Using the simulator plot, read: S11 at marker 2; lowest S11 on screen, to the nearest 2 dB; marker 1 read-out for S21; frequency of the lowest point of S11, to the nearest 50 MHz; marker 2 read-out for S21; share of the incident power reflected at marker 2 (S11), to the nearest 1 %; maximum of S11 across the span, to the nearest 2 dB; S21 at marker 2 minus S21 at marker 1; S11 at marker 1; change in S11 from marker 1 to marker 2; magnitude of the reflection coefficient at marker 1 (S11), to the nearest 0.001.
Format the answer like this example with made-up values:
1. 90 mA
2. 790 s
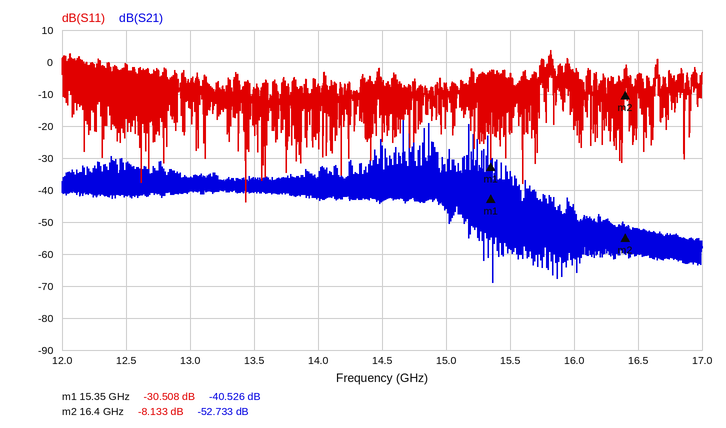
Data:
1. -8.133 dB
2. -44 dB
3. -40.526 dB
4. 13.45 GHz
5. -52.733 dB
6. 15 %
7. 4 dB
8. -12.207 dB
9. -30.508 dB
10. 22.375 dB
11. 0.030
